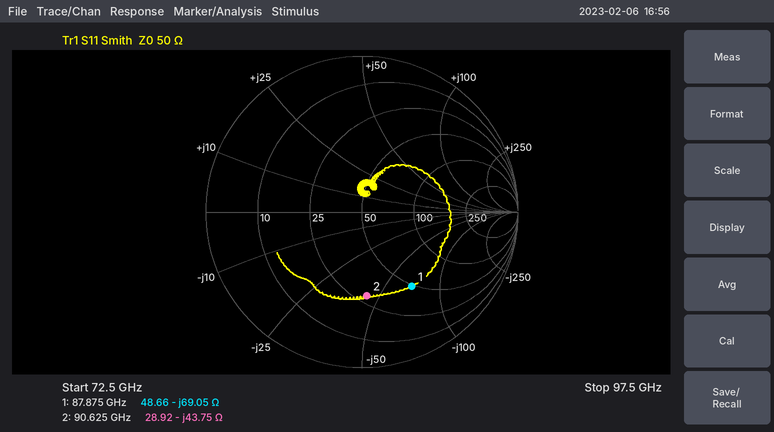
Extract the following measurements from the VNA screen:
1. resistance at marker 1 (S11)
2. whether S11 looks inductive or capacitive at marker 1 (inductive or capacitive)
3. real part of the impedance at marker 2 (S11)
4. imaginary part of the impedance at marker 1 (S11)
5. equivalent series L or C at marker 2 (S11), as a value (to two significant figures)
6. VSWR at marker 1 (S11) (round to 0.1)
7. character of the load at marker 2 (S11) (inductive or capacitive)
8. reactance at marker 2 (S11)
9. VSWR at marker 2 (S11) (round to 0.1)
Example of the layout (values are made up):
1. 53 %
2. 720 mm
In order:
1. 48.66 Ω
2. capacitive
3. 28.92 Ω
4. -69.05 Ω
5. 40 fF
6. 3.7
7. capacitive
8. -43.75 Ω
9. 3.3
